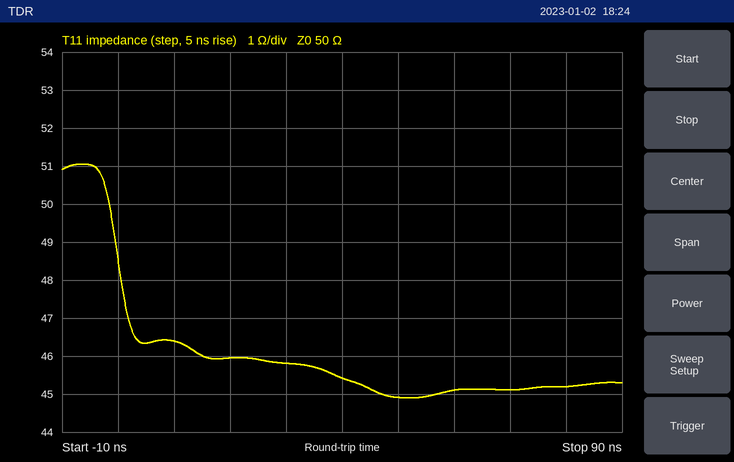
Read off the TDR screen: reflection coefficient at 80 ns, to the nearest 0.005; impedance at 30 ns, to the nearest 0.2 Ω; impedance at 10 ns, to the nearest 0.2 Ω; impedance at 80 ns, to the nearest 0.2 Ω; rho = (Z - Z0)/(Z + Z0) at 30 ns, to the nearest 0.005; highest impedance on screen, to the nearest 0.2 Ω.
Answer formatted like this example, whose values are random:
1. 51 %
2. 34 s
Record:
1. -0.050
2. 45.8 Ω
3. 46.4 Ω
4. 45.2 Ω
5. -0.045
6. 51.0 Ω
